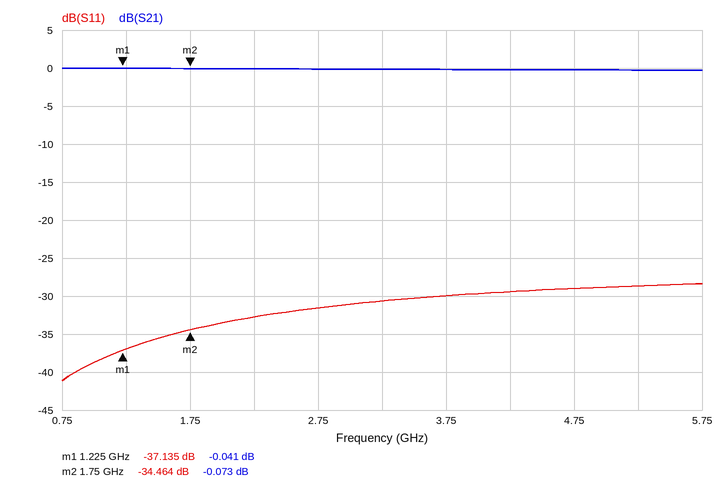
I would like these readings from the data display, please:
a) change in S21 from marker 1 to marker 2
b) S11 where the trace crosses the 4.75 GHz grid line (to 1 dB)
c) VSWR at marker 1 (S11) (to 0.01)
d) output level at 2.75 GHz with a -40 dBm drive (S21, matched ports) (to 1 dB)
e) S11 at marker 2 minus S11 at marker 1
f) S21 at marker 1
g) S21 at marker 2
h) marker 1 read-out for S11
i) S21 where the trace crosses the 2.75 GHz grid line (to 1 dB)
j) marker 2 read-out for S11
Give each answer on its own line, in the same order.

-0.032 dB
-29 dB
1.03
-40 dBm
2.671 dB
-0.041 dB
-0.073 dB
-37.135 dB
0 dB
-34.464 dB
